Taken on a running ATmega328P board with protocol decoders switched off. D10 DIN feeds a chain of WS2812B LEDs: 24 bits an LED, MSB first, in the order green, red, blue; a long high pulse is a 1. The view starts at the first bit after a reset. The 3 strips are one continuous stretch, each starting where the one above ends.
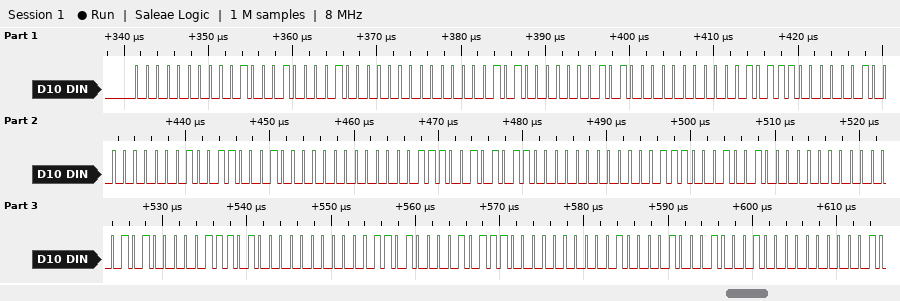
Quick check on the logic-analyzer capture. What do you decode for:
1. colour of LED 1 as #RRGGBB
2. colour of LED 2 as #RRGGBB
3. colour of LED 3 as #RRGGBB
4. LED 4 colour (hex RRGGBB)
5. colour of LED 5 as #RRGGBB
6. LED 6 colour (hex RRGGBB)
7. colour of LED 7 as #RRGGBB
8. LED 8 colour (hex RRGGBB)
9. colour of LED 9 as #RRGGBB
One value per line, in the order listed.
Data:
#220010
#28000A
#2E0004
#310100
#2B0700
#240E00
#1D1400
#171A00
#112100
